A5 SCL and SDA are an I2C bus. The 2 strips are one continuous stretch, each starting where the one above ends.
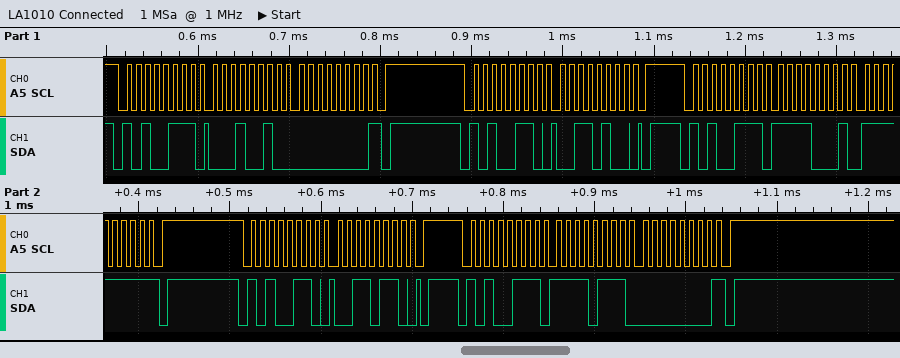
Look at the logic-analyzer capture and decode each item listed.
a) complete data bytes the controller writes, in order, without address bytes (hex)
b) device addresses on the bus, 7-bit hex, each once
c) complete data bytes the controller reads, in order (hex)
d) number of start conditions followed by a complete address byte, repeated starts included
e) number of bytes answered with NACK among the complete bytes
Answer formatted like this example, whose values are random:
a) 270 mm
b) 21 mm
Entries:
a) 34 36
b) 0x53
c) 12 00 F1 FF F7 00
d) 5
e) 3
